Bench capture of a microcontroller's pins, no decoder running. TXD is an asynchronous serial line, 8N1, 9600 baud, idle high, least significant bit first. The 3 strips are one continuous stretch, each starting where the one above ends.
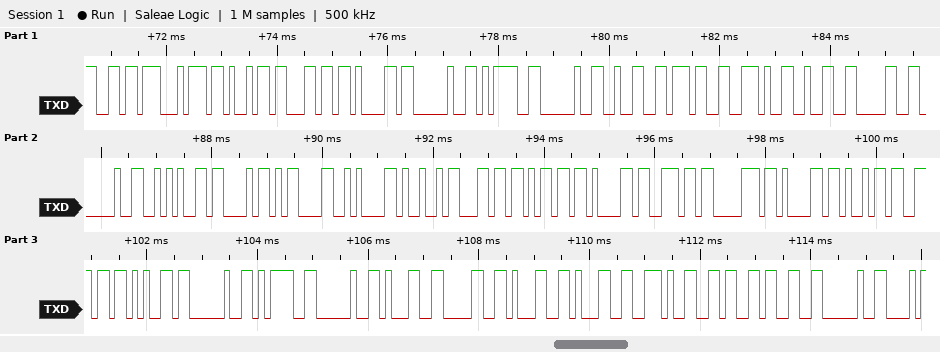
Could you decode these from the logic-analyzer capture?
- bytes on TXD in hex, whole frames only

B6 74 69 6C 61 20 3D 20 32 37 2E 32 30 20 2A 43 0D 0A 49 6C 6D 61 6E 70 61 69 6E 65 20 3D 20 31 30 31 31 2E 36 33 20
